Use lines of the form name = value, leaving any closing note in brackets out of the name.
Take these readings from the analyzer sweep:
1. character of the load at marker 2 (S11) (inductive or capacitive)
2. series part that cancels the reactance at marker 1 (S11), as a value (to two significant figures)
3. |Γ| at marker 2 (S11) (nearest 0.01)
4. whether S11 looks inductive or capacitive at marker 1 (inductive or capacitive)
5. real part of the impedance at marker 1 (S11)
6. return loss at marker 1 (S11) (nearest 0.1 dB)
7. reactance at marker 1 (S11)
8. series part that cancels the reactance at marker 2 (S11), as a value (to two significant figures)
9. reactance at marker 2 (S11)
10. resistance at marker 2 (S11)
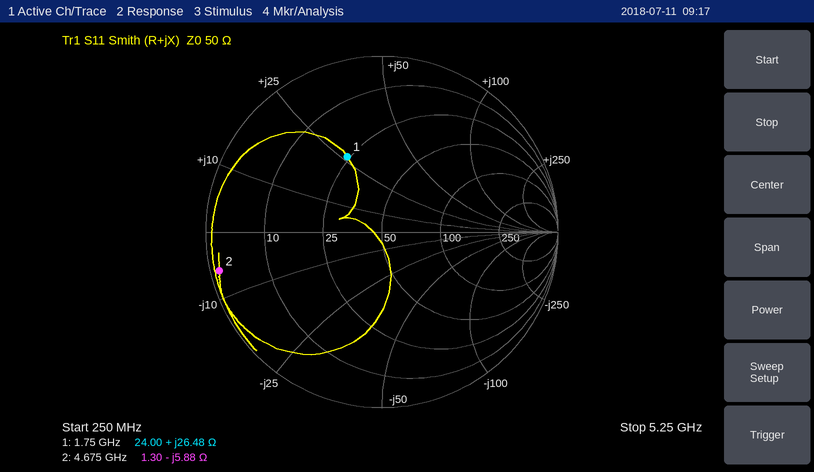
character of the load at marker 2 (S11) = capacitive
series part that cancels the reactance at marker 1 (S11), as a value = 3.4 pF
|Γ| at marker 2 (S11) = 0.95
whether S11 looks inductive or capacitive at marker 1 = inductive
real part of the impedance at marker 1 = 24.00 Ω
return loss at marker 1 (S11) = 6.5 dB
reactance at marker 1 = +26.48 Ω
series part that cancels the reactance at marker 2 (S11), as a value = 200 pH
reactance at marker 2 = -5.88 Ω
resistance at marker 2 = 1.30 Ω
